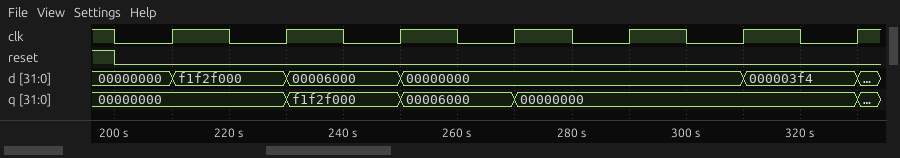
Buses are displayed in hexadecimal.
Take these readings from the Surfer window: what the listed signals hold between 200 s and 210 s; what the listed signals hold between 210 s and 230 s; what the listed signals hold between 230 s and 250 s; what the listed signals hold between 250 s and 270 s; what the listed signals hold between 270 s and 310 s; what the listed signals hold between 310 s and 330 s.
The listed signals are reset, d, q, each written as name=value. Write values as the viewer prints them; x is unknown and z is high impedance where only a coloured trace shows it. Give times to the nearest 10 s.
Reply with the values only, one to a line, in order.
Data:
reset=0, d=00000000, q=00000000
reset=0, d=f1f2f000, q=00000000
reset=0, d=00006000, q=f1f2f000
reset=0, d=00000000, q=00006000
reset=0, d=00000000, q=00000000
reset=0, d=000003f4, q=00000000
